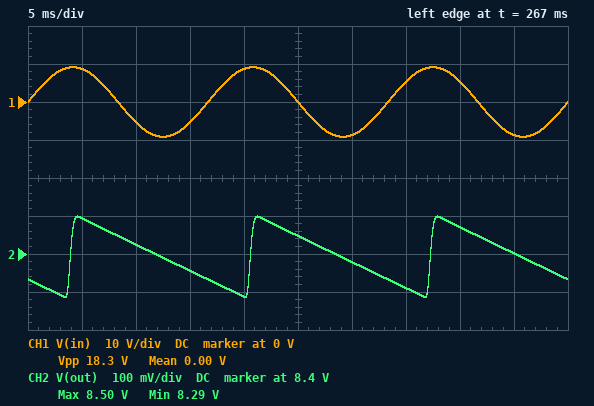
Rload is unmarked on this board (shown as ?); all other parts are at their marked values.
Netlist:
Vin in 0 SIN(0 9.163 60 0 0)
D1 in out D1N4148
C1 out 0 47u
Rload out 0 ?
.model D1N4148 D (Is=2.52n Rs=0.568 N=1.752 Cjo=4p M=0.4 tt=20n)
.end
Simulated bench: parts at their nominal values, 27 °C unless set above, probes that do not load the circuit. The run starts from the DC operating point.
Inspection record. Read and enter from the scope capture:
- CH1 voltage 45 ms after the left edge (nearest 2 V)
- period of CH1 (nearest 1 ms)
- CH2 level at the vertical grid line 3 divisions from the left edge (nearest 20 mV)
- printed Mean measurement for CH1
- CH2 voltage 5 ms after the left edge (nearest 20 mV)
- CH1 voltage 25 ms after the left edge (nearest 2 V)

-8 V
17 ms
8.36 V
0.00 V
8.50 V
0 V
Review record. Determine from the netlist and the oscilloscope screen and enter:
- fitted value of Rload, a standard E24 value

13 kΩ
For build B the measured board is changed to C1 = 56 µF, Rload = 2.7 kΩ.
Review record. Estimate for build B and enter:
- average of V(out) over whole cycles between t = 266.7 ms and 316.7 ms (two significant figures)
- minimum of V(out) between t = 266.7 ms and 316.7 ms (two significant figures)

8.1 V
7.7 V
